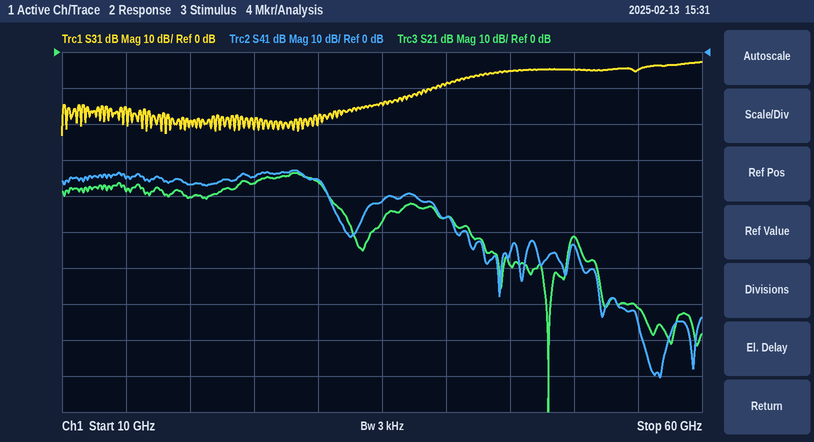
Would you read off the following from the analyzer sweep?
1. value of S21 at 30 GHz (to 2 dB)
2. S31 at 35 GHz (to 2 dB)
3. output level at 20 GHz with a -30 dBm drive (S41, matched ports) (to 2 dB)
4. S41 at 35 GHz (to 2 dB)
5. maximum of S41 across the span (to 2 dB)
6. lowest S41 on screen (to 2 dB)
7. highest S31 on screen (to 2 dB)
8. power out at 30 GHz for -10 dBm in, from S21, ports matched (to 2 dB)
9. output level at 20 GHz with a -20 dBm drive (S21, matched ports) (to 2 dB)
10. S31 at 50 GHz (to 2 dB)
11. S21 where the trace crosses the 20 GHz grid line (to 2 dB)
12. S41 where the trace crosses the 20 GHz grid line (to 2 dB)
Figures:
-36 dB
-14 dB
-66 dBm
-42 dB
-32 dB
-90 dB
-2 dB
-46 dBm
-60 dBm
-4 dB
-40 dB
-36 dB
